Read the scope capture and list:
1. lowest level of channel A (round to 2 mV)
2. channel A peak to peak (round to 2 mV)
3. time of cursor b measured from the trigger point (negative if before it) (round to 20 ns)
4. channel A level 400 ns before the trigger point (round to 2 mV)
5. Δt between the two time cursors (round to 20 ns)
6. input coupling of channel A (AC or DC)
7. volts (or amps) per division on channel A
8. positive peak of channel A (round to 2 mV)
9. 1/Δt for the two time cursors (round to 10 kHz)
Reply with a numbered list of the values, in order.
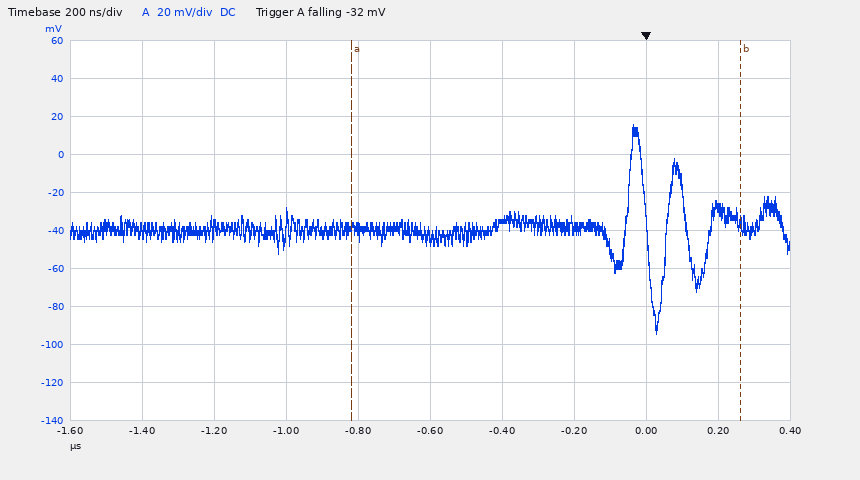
1. -94 mV
2. 110 mV
3. +260 ns
4. -34 mV
5. 1.08 µs
6. DC
7. 20 mV
8. 16 mV
9. 930 kHz
